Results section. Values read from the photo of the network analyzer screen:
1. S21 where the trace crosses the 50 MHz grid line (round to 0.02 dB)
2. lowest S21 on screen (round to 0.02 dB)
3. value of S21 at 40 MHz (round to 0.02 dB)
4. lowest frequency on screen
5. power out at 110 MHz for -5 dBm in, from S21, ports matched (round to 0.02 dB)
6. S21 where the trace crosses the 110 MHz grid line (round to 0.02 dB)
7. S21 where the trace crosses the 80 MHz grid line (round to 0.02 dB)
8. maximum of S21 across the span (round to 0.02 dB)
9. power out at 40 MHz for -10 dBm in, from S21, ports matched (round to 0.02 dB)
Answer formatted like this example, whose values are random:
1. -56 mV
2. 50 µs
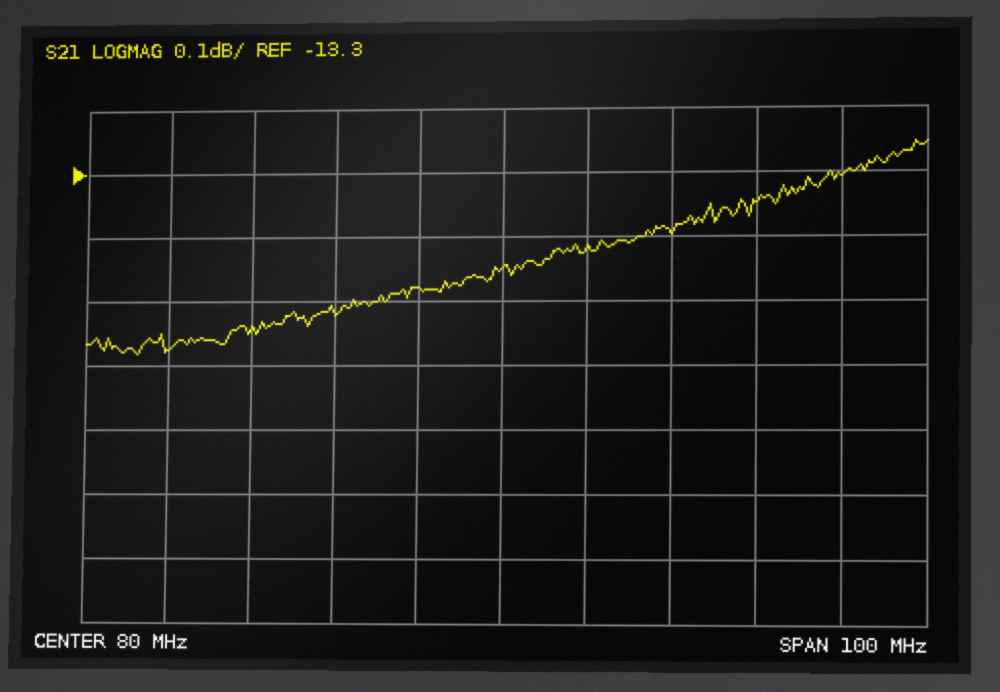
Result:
1. -13.54 dB
2. -13.58 dB
3. -13.58 dB
4. 30 MHz
5. -18.34 dBm
6. -13.34 dB
7. -13.44 dB
8. -13.26 dB
9. -23.58 dBm
